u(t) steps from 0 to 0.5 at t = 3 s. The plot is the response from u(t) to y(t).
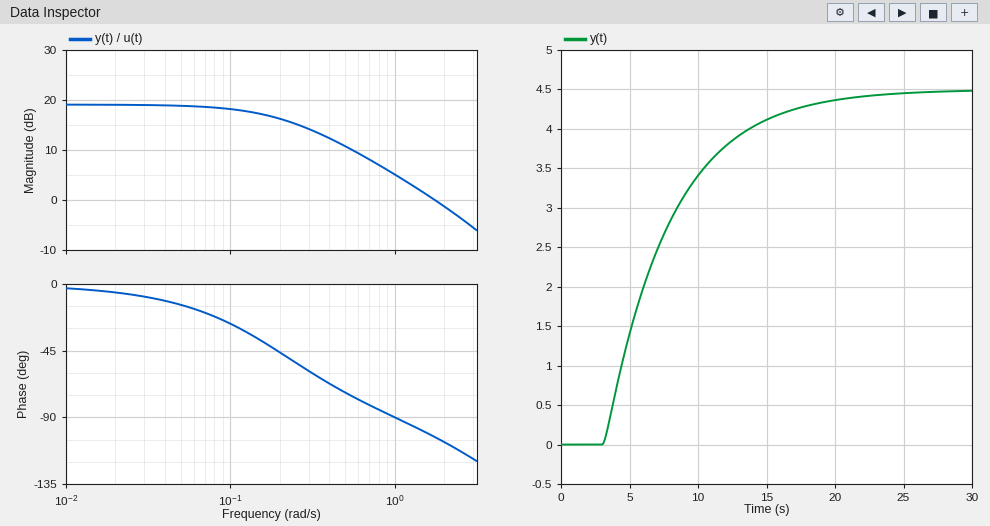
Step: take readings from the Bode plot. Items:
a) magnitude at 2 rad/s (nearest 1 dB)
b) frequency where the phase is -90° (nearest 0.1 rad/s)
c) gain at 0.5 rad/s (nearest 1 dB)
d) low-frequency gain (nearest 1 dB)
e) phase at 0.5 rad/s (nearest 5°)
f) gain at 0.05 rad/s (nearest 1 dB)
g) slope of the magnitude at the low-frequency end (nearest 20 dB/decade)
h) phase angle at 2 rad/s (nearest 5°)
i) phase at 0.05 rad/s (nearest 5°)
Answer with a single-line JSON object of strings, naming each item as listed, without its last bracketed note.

{"magnitude at 2 rad/s": "-1 dB", "frequency where the phase is -90°": "1.0 rad/s", "gain at 0.5 rad/s": "11 dB", "low-frequency gain": "19 dB", "phase at 0.5 rad/s": "-75°", "gain at 0.05 rad/s": "19 dB", "slope of the magnitude at the low-frequency end": "0 dB/decade", "phase angle at 2 rad/s": "-105°", "phase at 0.05 rad/s": "-15°"}
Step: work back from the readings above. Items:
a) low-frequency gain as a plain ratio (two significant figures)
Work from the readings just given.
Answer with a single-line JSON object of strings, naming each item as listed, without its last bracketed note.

{"low-frequency gain as a plain ratio": "8.9"}
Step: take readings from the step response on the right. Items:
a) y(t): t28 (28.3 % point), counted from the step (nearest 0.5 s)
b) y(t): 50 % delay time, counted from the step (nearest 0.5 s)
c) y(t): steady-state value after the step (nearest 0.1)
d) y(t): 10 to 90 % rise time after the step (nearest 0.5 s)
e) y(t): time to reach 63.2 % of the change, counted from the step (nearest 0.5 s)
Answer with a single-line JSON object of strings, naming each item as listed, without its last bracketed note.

{"y(t): t28 (28.3 % point), counted from the step": "2.0 s", "y(t): 50 % delay time, counted from the step": "3.5 s", "y(t): steady-state value after the step": "4.5", "y(t): 10 to 90 % rise time after the step": "10.5 s", "y(t): time to reach 63.2 % of the change, counted from the step": "5.0 s"}
